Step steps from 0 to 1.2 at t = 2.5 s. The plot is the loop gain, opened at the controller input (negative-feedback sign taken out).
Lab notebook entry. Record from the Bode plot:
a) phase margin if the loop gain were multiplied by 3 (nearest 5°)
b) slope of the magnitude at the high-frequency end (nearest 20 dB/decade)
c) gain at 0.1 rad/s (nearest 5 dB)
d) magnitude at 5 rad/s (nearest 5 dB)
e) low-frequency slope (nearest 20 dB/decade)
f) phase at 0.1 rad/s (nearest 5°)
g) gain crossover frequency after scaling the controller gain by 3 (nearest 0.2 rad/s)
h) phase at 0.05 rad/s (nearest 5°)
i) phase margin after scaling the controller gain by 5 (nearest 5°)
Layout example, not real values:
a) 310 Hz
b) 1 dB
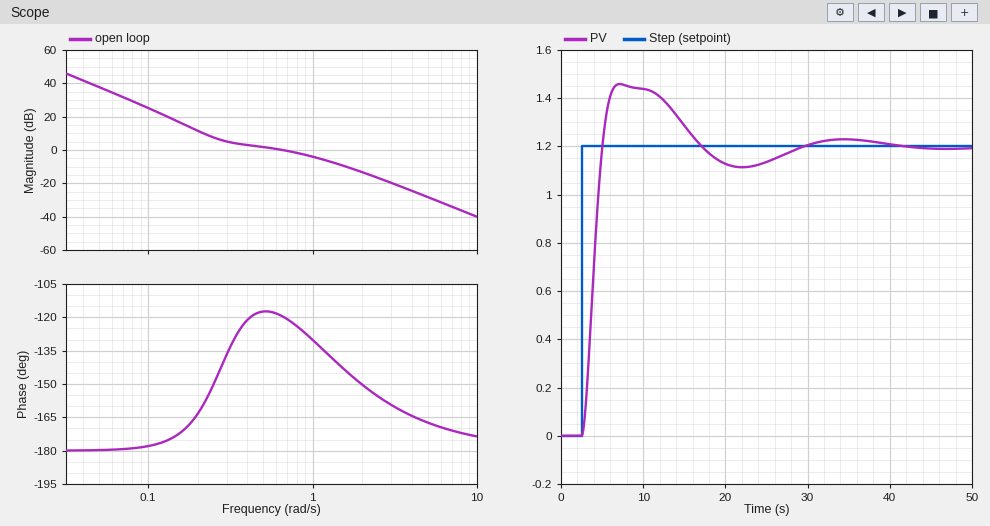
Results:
a) 35°
b) -40 dB/decade
c) 25 dB
d) -30 dB
e) -40 dB/decade
f) -180°
g) 1.6 rad/s
h) -180°
i) 30°
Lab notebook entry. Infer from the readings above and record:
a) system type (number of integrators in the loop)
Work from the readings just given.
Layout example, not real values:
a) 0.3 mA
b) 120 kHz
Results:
a) 2
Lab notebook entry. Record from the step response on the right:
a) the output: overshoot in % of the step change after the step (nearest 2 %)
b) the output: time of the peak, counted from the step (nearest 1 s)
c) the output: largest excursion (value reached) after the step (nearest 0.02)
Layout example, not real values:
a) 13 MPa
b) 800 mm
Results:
a) 22 %
b) 5 s
c) 1.46
